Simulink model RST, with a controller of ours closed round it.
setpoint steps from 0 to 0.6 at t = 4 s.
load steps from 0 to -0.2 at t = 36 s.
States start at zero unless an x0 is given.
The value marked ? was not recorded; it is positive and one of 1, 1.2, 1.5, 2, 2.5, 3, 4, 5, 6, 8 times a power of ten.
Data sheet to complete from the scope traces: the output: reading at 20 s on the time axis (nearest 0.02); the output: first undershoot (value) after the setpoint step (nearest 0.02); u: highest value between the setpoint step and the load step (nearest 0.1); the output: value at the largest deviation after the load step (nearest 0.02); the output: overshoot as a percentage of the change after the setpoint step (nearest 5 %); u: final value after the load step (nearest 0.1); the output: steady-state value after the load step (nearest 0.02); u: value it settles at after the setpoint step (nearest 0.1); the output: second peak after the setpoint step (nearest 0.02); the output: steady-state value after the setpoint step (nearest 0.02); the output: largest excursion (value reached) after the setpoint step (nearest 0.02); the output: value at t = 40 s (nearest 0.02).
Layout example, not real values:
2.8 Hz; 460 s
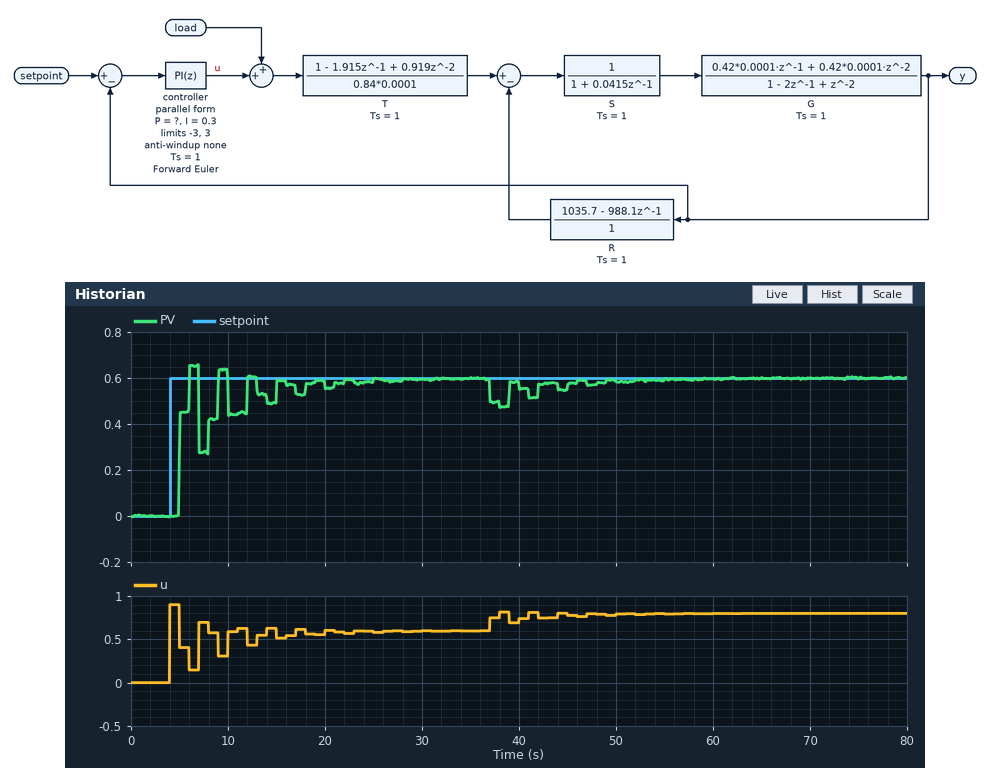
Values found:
0.56; 0.28; 0.9; 0.48; 10 %; 0.8; 0.60; 0.6; 0.64; 0.60; 0.66; 0.56
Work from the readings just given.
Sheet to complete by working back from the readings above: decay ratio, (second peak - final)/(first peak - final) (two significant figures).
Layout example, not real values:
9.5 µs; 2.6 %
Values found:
0.67
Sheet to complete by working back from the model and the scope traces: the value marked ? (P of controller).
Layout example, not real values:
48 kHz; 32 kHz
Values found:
1.5
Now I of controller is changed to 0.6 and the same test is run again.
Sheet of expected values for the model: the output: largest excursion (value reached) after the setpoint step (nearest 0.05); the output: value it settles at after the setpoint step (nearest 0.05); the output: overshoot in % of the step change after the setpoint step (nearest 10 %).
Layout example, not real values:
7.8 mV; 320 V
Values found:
0.75; 0.60; 20 %
